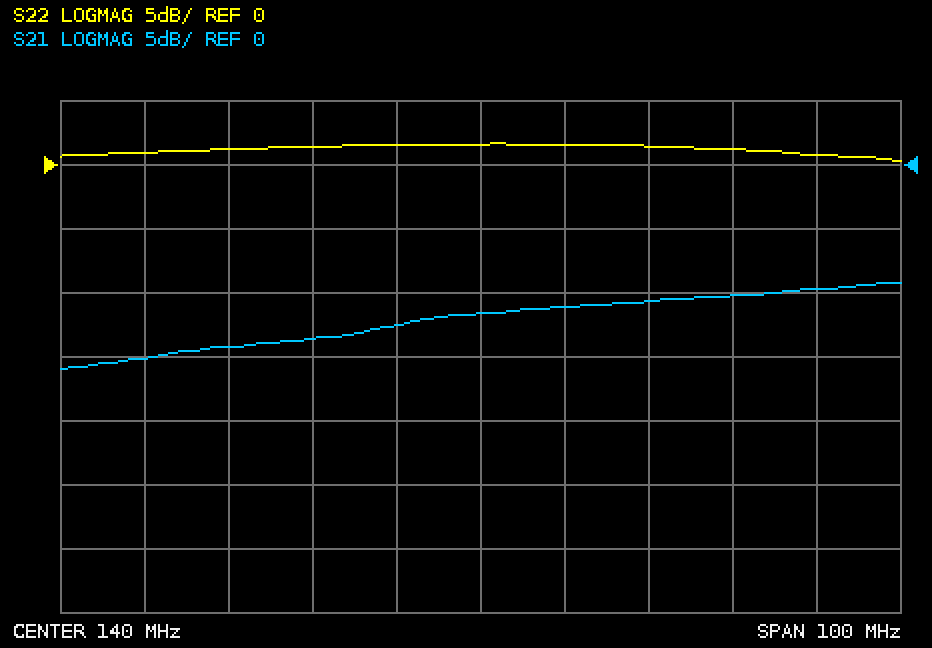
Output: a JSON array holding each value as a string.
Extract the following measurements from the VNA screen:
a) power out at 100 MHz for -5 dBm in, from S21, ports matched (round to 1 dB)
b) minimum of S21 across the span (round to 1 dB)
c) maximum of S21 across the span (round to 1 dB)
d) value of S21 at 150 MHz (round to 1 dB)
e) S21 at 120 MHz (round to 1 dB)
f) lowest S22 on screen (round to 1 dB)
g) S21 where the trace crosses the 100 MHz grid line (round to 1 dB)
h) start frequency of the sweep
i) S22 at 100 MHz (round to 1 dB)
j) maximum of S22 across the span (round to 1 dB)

["-20 dBm", "-16 dB", "-9 dB", "-11 dB", "-14 dB", "0 dB", "-15 dB", "90 MHz", "1 dB", "2 dB"]
